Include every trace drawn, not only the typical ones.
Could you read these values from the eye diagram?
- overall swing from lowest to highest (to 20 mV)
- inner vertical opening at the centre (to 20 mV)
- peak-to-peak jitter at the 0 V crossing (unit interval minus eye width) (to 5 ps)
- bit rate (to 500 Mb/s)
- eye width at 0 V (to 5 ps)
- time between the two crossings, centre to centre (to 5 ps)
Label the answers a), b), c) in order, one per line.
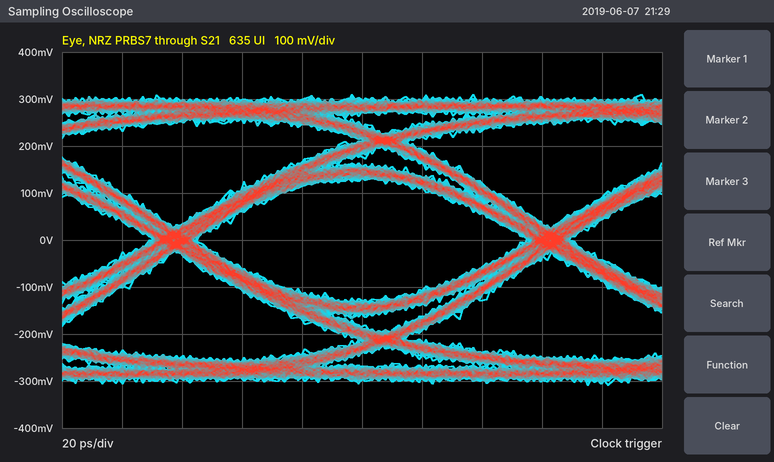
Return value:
a) 620 mV
b) 260 mV
c) 15 ps
d) 8.0 Gb/s
e) 110 ps
f) 125 ps
